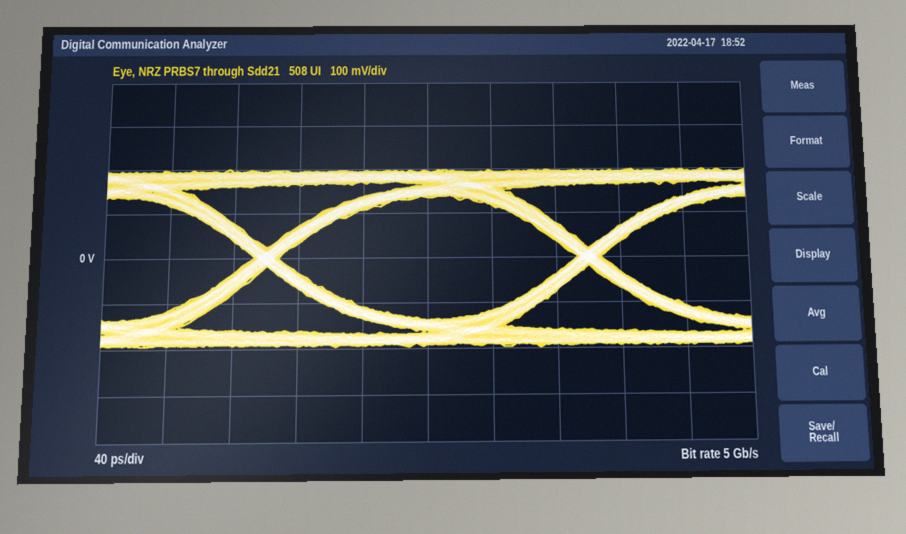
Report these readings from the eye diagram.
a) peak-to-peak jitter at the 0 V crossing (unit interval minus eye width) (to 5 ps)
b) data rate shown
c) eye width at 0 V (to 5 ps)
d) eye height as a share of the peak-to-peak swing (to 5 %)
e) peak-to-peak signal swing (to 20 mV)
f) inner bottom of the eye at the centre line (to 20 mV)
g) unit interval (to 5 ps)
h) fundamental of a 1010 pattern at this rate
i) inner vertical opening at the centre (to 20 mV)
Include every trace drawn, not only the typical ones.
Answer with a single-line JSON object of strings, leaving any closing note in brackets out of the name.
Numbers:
{"peak-to-peak jitter at the 0 V crossing (unit interval minus eye width)": "15 ps", "data rate shown": "5 Gb/s", "eye width at 0 V": "185 ps", "eye height as a share of the peak-to-peak swing": "70 %", "peak-to-peak signal swing": "400 mV", "inner bottom of the eye at the centre line": "-140 mV", "unit interval": "200 ps", "fundamental of a 1010 pattern at this rate": "2.5 GHz", "inner vertical opening at the centre": "280 mV"}
